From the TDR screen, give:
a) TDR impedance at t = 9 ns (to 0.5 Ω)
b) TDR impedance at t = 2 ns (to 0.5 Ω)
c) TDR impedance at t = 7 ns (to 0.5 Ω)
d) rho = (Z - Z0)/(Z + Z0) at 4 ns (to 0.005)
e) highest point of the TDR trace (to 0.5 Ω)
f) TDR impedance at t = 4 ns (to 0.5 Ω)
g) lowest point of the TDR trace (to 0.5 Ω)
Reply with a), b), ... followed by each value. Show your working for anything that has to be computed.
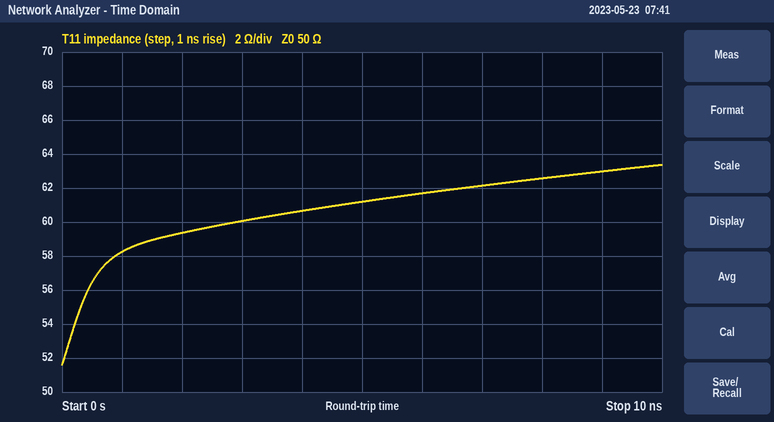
a) 63.0 Ω
b) 59.5 Ω
c) 62.0 Ω
d) (60.5 − 50)/(60.5 + 50) ≈ +0.095
e) 63.5 Ω
f) 60.5 Ω
g) 51.5 Ω
